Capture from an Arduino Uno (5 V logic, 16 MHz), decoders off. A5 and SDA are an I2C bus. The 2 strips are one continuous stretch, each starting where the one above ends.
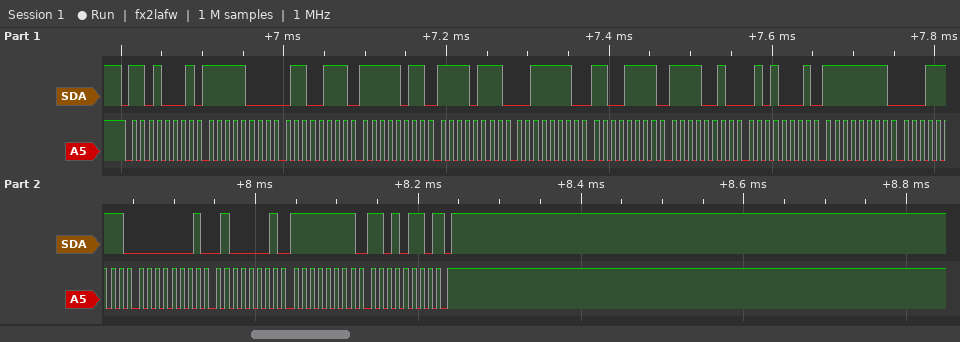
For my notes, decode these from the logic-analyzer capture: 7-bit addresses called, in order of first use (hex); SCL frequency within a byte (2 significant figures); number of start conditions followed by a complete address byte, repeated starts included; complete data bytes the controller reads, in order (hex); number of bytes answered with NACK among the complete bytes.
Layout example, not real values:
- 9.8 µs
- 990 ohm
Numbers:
- 0x68
- 100 kHz
- 1
- F8 67 FB F7 3E CF F2 51 FF 1F 01 41 FF D6
- 1
